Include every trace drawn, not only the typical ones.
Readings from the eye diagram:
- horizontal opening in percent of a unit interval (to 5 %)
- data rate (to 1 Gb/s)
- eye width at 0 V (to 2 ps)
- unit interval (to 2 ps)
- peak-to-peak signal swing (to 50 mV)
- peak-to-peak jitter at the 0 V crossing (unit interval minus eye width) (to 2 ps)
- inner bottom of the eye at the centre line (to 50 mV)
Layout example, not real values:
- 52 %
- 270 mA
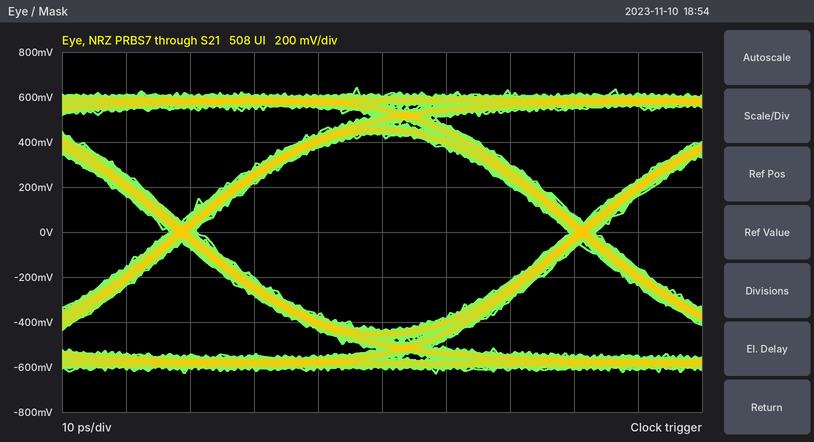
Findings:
- 95 %
- 16 Gb/s
- 58 ps
- 62 ps
- 1.25 V
- 4 ps
- -450 mV
